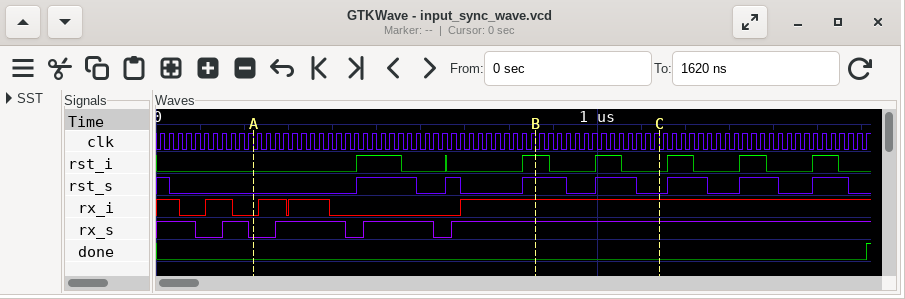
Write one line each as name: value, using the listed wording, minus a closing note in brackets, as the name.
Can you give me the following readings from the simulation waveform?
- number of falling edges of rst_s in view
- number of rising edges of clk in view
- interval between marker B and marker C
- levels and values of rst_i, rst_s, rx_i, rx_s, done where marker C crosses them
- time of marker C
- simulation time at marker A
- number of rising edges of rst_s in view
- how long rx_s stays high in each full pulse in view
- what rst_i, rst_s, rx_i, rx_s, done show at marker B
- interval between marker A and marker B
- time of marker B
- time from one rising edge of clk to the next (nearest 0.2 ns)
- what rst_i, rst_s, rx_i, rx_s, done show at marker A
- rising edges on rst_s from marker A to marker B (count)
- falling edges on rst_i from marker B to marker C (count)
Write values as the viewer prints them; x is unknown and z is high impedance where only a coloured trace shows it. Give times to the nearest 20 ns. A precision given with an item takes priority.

number of falling edges of rst_s in view: 8
number of rising edges of clk in view: 81
interval between marker B and marker C: 280 ns
levels and values of rst_i, rst_s, rx_i, rx_s, done where marker C crosses them: rst_i=0, rst_s=0, rx_i=1, rx_s=1, done=0
time of marker C: 1140 ns
simulation time at marker A: 220 ns
number of rising edges of rst_s in view: 7
how long rx_s stays high in each full pulse in view: 60 ns, 160 ns, 160 ns
what rst_i, rst_s, rx_i, rx_s, done show at marker B: rst_i=1, rst_s=1, rx_i=1, rx_s=1, done=0
interval between marker A and marker B: 640 ns
time of marker B: 860 ns
time from one rising edge of clk to the next: 20 ns
what rst_i, rst_s, rx_i, rx_s, done show at marker A: rst_i=0, rst_s=0, rx_i=0, rx_s=0, done=0
rising edges on rst_s from marker A to marker B: 3
falling edges on rst_i from marker B to marker C: 2
